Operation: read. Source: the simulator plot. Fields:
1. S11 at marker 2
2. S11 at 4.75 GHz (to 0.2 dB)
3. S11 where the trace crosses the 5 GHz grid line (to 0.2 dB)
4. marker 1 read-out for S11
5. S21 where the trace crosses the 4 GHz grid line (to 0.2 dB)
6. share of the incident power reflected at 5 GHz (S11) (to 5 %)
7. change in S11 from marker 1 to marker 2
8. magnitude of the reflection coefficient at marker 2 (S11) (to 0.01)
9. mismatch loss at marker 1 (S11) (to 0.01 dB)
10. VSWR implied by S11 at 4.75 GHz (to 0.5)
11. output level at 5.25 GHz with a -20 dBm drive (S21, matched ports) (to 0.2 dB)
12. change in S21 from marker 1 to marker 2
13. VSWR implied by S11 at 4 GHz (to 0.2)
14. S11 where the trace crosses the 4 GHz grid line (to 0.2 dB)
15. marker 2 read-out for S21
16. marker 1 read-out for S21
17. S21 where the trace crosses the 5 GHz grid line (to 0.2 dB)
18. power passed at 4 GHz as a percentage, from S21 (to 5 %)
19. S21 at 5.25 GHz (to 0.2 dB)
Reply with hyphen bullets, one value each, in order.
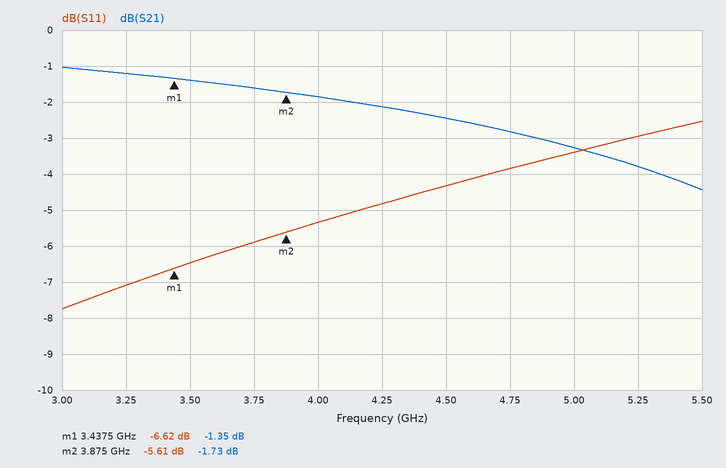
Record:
- -5.61 dB
- -3.8 dB
- -3.4 dB
- -6.62 dB
- -1.8 dB
- 45 %
- 1.01 dB
- 0.52
- 1.07 dB
- 4.5
- -23.8 dBm
- -0.38 dB
- 3.4
- -5.4 dB
- -1.73 dB
- -1.35 dB
- -3.2 dB
- 65 %
- -3.8 dB
